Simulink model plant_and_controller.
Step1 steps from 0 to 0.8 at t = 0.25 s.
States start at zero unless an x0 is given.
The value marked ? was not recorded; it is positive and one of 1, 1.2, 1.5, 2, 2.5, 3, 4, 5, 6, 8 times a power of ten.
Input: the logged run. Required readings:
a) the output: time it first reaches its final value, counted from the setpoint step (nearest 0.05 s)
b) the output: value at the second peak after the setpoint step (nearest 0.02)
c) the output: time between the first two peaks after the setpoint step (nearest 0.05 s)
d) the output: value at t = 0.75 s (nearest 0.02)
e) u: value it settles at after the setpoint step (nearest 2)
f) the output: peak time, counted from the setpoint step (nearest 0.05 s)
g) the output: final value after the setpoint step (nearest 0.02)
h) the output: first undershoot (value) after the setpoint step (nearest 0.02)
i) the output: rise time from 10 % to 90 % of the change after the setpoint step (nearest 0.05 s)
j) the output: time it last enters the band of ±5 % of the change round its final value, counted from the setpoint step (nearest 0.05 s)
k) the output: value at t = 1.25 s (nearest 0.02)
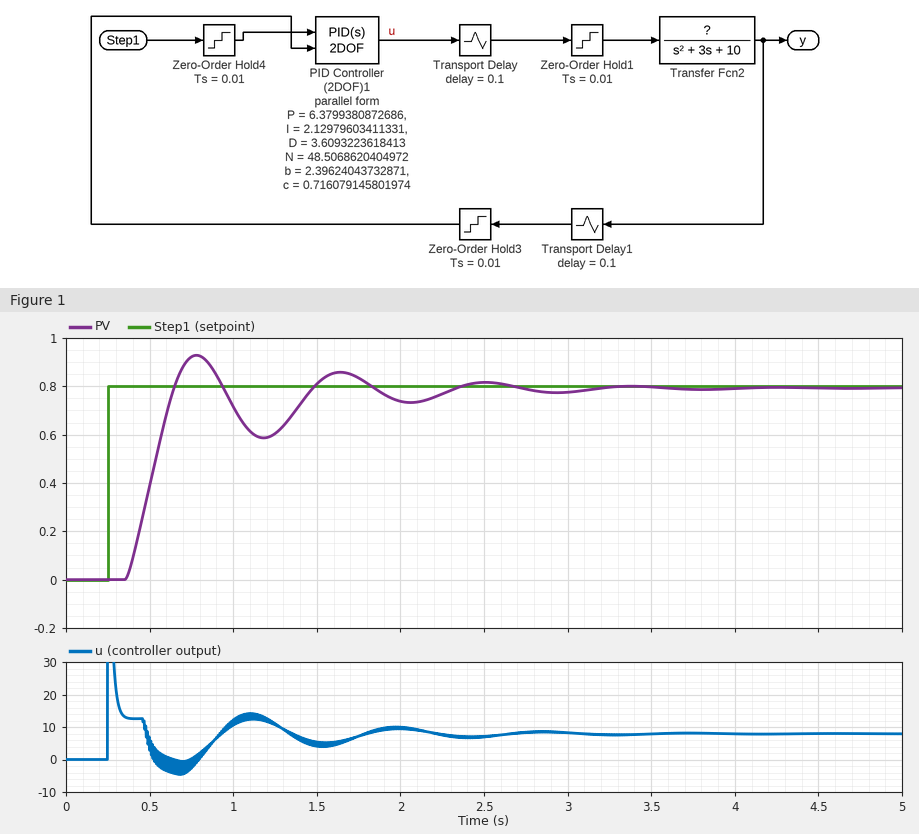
0.40 s
0.86
0.85 s
0.92
8
0.55 s
0.80
0.58
0.20 s
1.95 s
0.60
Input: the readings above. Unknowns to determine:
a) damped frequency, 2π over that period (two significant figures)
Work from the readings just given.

7.4 rad/s
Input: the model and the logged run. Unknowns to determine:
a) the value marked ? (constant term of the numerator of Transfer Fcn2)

1
